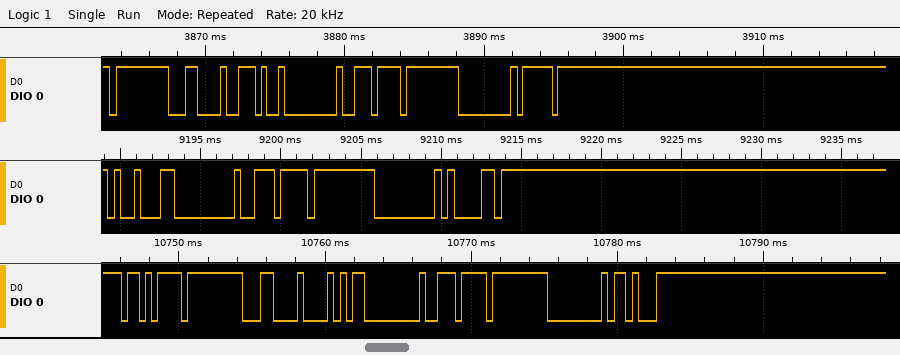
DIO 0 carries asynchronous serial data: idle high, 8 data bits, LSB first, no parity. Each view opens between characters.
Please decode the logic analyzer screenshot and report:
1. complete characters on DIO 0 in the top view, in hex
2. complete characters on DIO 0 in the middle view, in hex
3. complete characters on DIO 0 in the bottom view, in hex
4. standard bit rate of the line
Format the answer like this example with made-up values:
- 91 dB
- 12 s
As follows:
- FF, 0C, 2E, 00, EE, FF, 00, DF
- 89, 00, EE, FF, 00, 61
- EB, FF, 0C, A8, 00, EE, FF, 00, 8B
- 2400 baud
